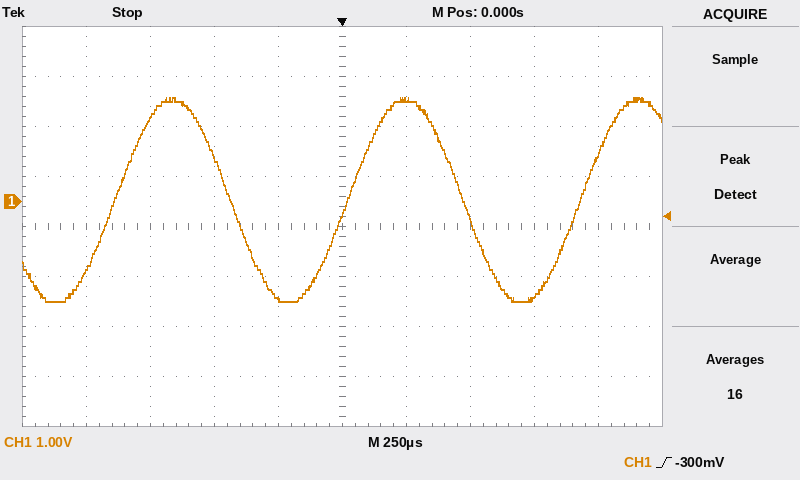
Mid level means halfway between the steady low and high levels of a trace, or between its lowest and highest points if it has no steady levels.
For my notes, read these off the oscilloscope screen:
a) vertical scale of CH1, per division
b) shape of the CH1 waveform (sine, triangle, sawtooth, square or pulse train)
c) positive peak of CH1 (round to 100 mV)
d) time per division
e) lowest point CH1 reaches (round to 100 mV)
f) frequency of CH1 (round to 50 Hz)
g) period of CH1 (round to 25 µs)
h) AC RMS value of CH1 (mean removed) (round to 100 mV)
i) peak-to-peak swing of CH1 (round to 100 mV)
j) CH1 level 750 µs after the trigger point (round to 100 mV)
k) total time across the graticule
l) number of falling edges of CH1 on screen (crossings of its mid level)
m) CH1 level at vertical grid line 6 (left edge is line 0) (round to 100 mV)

1 V
sine
2.1 V
250 µs
-2.0 V
1.10 kHz
900 µs
1.4 V
4.1 V
-1.9 V
2.5 ms
2
2.0 V
